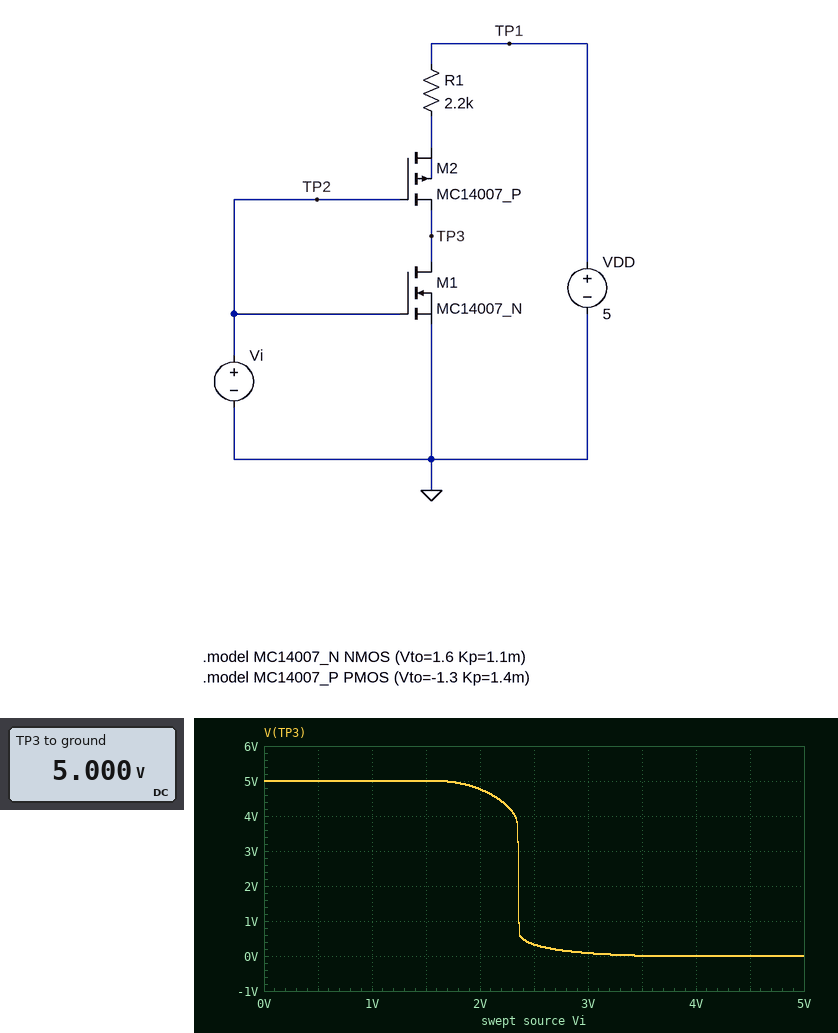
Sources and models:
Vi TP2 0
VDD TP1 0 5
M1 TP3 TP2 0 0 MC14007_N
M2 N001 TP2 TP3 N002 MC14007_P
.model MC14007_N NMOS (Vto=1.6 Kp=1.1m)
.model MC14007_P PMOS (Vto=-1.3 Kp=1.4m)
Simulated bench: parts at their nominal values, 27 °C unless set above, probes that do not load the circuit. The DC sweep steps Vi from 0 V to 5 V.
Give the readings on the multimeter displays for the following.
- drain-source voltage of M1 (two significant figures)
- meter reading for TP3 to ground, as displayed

5.0 V
5.000 V
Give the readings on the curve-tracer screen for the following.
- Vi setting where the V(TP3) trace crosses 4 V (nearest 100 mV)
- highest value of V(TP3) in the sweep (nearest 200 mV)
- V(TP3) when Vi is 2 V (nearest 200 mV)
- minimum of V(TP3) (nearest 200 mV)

2.3 V
5.0 V
4.8 V
0 V
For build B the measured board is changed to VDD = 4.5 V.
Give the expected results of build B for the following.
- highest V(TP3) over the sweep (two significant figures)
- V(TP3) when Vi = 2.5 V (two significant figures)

4.5 V
140 mV
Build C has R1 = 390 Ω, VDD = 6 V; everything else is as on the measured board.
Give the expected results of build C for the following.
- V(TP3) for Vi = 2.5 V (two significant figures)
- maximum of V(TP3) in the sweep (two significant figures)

5.7 V
6.0 V
